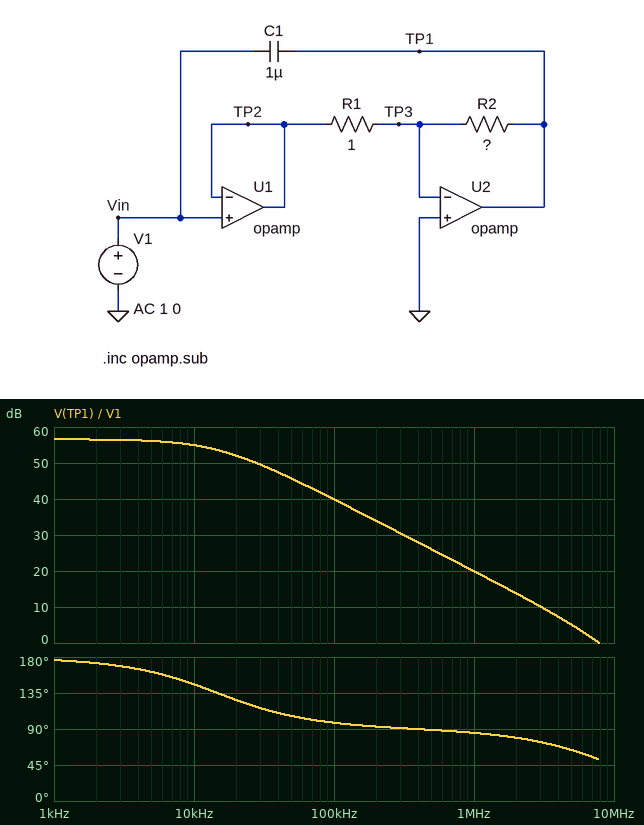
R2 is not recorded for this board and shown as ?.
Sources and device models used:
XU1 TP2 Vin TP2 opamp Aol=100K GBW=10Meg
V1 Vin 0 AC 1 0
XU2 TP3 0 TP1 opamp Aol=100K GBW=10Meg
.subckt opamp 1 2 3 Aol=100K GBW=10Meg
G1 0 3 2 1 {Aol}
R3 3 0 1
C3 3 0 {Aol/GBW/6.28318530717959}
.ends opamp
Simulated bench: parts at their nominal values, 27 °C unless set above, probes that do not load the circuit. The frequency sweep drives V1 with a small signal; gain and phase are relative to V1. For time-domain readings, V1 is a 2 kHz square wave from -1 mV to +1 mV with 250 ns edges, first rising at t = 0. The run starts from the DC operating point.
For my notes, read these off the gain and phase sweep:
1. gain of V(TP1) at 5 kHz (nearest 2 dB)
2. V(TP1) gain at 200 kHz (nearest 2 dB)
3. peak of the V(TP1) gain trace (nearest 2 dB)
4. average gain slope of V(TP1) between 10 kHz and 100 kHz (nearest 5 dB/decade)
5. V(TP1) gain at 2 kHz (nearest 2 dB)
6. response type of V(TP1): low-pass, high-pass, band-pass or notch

56 dB
34 dB
56 dB
-15 dB/decade
56 dB
low-pass
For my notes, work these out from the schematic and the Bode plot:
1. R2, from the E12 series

680 Ω
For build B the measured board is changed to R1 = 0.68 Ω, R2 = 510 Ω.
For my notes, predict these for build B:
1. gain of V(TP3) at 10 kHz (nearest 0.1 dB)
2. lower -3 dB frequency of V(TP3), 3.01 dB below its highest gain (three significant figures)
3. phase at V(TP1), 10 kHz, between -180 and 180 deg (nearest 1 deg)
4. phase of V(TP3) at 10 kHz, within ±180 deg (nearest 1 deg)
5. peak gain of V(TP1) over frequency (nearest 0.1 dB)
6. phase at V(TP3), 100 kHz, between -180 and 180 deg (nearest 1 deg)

-4.5 dB
13.4 kHz
143 deg
53 deg
57.4 dB
7 deg
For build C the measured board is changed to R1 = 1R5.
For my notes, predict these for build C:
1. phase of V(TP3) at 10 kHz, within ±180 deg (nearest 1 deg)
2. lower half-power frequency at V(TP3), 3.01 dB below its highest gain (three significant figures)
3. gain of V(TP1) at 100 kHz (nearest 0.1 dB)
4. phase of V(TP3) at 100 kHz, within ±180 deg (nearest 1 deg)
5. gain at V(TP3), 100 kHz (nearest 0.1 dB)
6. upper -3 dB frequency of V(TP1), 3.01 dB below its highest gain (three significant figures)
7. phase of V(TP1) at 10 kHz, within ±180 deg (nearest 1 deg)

65 deg
22.0 kHz
39.8 dB
12 deg
-0.2 dB
22.1 kHz
156 deg
